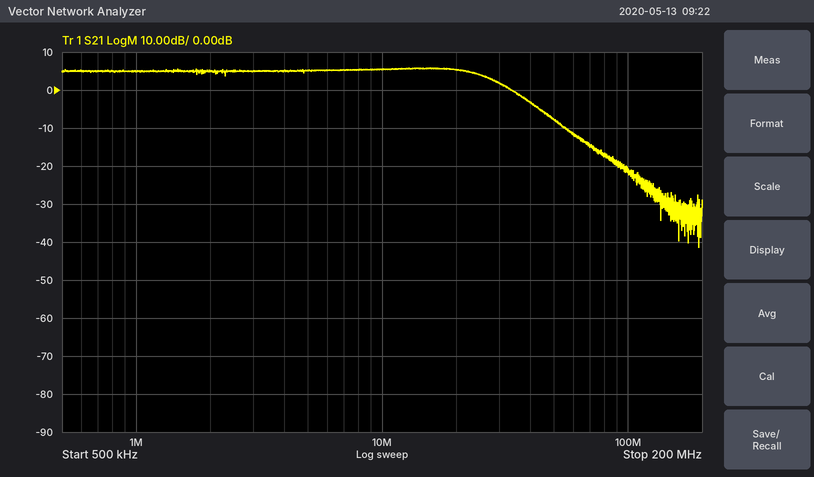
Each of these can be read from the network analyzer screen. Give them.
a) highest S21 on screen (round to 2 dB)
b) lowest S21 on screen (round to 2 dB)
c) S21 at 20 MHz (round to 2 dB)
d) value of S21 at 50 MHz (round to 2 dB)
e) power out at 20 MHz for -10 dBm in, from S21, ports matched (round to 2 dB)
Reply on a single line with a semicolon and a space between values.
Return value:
6 dB; -42 dB; 6 dB; -8 dB; -4 dBm
